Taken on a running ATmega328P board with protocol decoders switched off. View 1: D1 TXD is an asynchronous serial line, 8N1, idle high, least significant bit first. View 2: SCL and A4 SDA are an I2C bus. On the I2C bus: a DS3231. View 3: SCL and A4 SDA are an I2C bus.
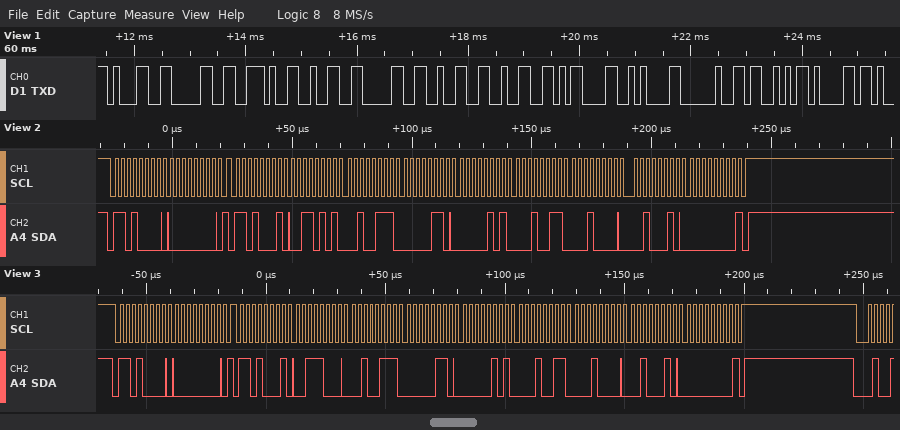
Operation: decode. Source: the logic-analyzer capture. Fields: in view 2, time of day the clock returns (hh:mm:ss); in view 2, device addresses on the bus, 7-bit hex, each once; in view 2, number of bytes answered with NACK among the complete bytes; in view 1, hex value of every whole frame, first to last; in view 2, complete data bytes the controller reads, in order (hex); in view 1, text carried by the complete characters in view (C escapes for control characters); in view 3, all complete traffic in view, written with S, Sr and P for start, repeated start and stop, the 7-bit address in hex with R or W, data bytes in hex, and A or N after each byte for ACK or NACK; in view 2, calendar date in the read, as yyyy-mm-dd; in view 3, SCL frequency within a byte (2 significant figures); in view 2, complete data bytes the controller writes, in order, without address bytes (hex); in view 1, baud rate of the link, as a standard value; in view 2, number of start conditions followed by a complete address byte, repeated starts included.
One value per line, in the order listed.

06:27:35
0x68
1
0x31 0x30 0x2E 0x32 0x30 0x32 0x32 0x0D 0x0A 0x20 0x53 0x61
35 27 06 05 13 10 22 00
"10.2022\r\n Sa"
S 68W A 00 A Sr 68R A 38 A 27 A 06 A 05 A 13 A 10 A 22 A 00 N P
2022-10-13
400 kHz
00
9600 baud
2
